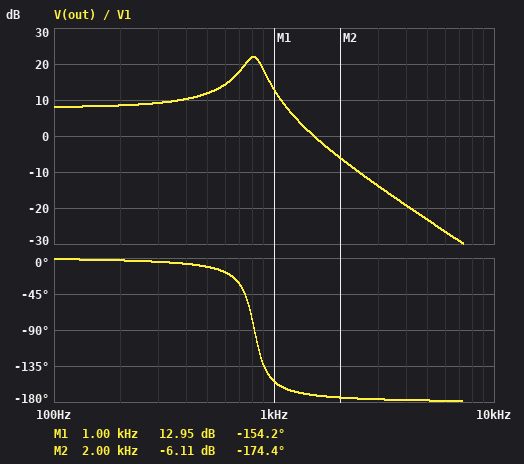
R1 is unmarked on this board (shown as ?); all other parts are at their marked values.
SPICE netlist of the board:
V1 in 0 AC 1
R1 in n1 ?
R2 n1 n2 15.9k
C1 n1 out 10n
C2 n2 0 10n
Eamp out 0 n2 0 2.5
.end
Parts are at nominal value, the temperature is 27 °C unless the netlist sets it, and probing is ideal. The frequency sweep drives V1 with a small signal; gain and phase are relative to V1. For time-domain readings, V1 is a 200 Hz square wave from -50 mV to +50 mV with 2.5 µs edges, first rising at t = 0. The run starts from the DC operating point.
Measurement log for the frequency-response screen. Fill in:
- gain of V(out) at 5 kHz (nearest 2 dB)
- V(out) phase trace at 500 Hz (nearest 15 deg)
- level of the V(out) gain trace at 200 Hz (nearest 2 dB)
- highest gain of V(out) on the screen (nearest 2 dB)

-24 dB
-15 deg
8 dB
22 dB
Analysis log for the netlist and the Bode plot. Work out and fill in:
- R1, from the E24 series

24 kΩ
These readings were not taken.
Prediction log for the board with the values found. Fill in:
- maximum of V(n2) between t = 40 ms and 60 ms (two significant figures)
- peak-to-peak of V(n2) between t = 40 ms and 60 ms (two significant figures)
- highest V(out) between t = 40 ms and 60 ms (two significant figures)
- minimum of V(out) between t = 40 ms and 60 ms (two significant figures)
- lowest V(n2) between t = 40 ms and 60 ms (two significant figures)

110 mV
210 mV
270 mV
-270 mV
-110 mV
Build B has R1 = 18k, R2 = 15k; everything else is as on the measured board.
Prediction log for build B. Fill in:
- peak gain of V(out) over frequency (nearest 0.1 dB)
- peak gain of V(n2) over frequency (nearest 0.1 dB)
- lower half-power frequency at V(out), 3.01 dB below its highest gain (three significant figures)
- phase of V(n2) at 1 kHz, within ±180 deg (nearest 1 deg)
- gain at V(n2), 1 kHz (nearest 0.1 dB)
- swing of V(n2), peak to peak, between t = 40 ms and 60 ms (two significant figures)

16.9 dB
8.9 dB
734 Hz
-100 deg
8.3 dB
220 mV
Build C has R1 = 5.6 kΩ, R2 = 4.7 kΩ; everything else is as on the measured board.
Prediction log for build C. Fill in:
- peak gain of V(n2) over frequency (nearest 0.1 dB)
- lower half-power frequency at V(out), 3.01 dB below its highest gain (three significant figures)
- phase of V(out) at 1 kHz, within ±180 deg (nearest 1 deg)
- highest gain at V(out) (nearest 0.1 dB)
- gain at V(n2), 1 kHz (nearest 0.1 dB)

8.8 dB
2.34 kHz
-8 deg
16.7 dB
0.9 dB
